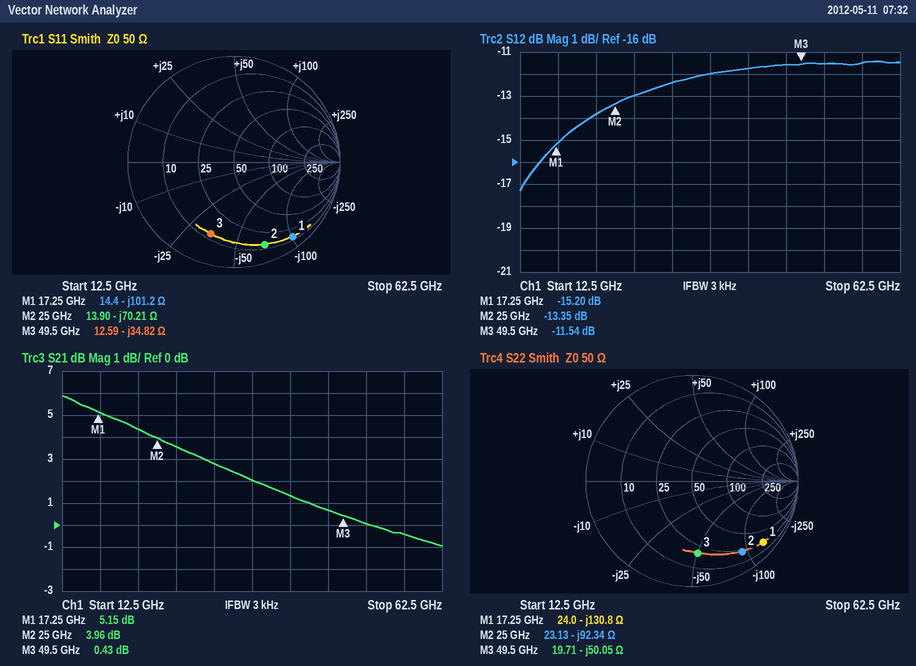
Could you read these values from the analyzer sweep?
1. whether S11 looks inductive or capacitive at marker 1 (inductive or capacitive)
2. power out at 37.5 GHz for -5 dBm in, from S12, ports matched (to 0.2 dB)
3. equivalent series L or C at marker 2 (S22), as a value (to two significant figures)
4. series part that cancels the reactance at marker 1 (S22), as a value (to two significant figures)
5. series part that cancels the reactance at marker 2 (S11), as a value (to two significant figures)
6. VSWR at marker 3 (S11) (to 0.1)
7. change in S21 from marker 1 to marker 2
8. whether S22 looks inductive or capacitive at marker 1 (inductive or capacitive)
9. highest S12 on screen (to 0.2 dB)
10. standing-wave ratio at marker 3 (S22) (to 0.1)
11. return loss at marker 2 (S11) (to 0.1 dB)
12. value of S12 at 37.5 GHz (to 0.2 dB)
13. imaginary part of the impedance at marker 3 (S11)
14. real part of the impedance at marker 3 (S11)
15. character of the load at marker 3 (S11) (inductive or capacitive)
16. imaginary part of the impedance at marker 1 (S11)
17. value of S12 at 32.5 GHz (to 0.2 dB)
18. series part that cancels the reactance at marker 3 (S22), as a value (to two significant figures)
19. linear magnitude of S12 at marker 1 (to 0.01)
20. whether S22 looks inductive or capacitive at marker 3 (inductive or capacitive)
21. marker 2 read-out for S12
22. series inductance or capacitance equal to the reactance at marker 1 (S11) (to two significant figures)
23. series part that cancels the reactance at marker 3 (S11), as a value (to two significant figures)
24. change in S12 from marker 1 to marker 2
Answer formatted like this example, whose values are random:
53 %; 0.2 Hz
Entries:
capacitive; -17.0 dBm; 69 fF; 1.2 nH; 450 pH; 6.0; -1.19 dB; capacitive; -11.4 dB; 5.3; 1.6 dB; -12.0 dB; -34.82 Ω; 12.59 Ω; capacitive; -101.2 Ω; -12.4 dB; 160 pH; 0.17; capacitive; -13.35 dB; 91 fF; 110 pH; 1.85 dB
